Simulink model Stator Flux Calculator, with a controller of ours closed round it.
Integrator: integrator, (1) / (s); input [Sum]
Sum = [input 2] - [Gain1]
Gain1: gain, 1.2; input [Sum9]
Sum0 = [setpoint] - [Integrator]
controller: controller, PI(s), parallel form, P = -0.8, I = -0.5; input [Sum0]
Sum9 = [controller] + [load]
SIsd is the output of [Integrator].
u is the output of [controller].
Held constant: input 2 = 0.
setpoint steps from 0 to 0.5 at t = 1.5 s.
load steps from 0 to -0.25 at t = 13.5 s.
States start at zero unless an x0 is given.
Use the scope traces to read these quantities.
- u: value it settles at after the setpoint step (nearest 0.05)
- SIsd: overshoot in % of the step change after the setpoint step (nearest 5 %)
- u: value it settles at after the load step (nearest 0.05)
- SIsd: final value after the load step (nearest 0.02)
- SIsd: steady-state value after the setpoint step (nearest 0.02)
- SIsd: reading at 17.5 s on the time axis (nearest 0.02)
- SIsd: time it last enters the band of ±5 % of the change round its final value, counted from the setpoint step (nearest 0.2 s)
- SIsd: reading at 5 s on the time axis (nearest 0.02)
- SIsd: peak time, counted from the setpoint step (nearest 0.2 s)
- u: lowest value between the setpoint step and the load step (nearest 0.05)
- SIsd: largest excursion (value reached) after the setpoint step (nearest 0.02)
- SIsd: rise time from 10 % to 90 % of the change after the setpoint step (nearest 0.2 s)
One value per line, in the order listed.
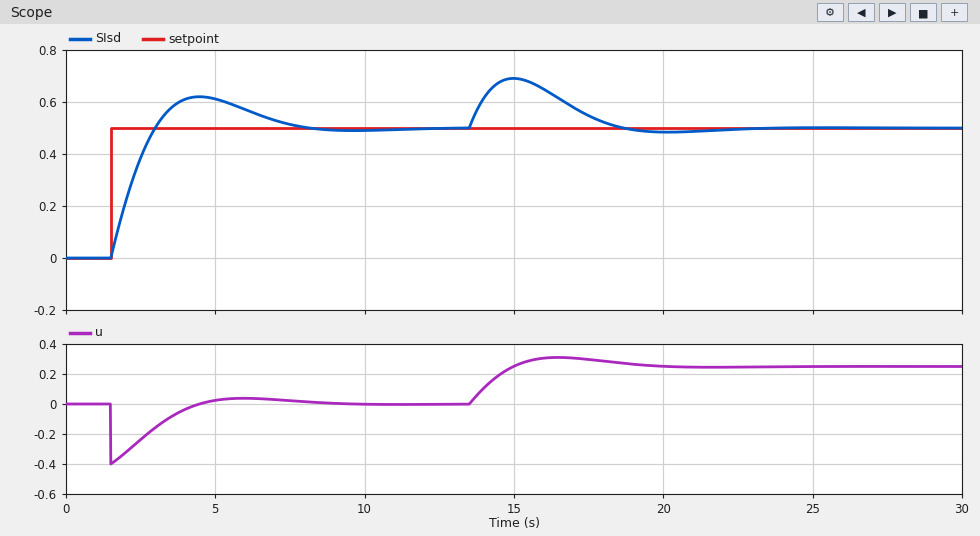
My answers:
0.00
25 %
0.25
0.50
0.50
0.54
5.6 s
0.62
3.0 s
-0.40
0.62
1.2 s
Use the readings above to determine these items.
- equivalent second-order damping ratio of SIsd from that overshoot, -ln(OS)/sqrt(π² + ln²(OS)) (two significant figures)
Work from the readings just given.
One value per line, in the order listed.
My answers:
0.40
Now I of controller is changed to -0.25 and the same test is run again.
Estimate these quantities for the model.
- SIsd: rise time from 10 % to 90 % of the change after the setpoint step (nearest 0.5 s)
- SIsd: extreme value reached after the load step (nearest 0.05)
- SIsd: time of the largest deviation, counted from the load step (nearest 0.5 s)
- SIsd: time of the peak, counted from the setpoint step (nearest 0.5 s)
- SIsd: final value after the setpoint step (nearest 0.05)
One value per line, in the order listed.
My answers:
1.5 s
0.70
2.0 s
4.0 s
0.50
